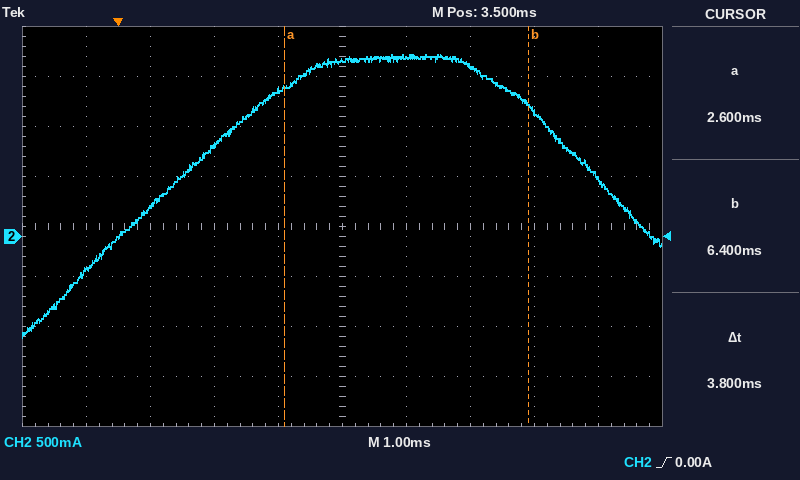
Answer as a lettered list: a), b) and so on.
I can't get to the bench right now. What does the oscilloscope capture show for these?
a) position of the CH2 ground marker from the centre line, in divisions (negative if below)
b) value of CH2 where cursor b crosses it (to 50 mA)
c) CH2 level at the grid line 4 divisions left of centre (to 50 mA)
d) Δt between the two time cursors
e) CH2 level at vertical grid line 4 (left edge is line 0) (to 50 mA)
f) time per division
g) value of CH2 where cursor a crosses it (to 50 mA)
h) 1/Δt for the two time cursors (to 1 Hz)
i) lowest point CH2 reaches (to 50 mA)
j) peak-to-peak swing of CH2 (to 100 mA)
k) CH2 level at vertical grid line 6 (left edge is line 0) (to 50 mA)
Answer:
a) -0.2 div
b) 1.30 A
c) -350 mA
d) 3.8 ms
e) 1.45 A
f) 1 ms
g) 1.50 A
h) 263 Hz
i) -1.00 A
j) 2.80 A
k) 1.80 A
